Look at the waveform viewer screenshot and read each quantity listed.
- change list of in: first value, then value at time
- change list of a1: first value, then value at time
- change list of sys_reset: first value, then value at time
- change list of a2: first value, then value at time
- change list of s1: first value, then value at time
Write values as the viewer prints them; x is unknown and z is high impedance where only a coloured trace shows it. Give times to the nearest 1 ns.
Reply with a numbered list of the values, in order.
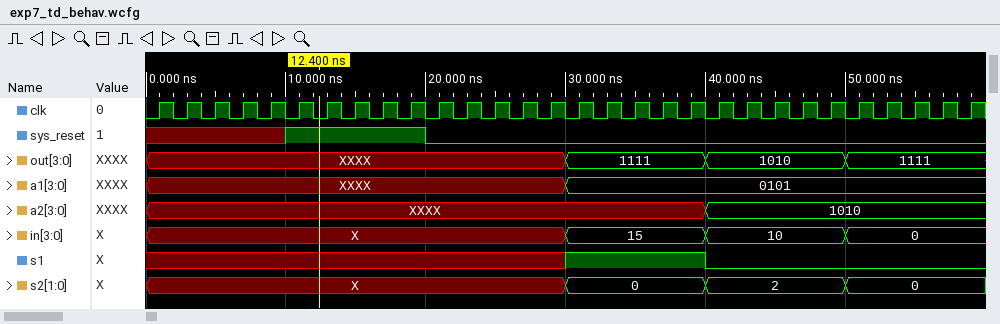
1. X, 15 at 30 ns, 10 at 40 ns, 0 at 50 ns
2. XXXX, 0101 at 30 ns
3. x, 1 at 10 ns, 0 at 20 ns
4. XXXX, 1010 at 40 ns
5. x, 1 at 30 ns, 0 at 40 ns
